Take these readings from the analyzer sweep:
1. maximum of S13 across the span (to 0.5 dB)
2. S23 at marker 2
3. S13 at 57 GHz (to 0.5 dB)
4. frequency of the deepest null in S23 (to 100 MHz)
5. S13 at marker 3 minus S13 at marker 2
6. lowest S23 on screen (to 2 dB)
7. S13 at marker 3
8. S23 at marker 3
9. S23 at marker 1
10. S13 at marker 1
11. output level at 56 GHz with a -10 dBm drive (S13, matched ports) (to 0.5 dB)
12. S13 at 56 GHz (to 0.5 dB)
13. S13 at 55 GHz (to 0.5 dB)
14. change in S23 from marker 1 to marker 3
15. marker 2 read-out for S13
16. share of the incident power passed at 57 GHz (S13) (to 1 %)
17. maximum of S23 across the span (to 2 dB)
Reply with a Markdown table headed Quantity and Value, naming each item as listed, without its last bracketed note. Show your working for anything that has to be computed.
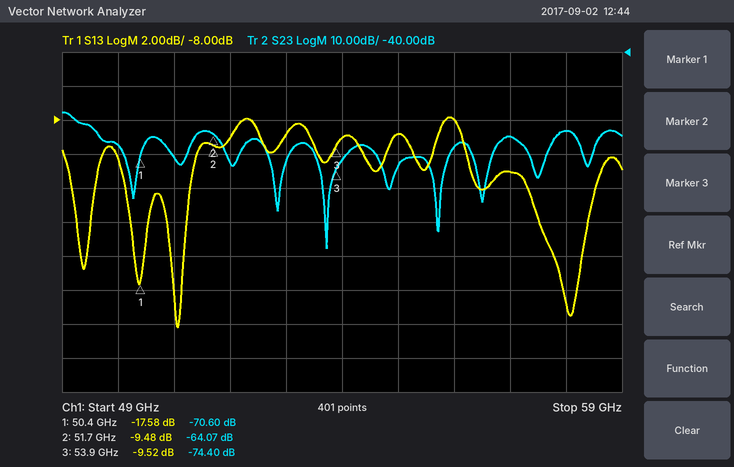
| Quantity | Value |
|---|---|
| maximum of S13 across the span | -8.0 dB |
| S23 at marker 2 | -64.07 dB |
| S13 at 57 GHz | -11.0 dB |
| frequency of the deepest null in S23 | 53.7 GHz |
| S13 at marker 3 minus S13 at marker 2 | -9.52 − (-9.48) = -0.04 dB |
| lowest S23 on screen | -98 dB |
| S13 at marker 3 | -9.52 dB |
| S23 at marker 3 | -74.40 dB |
| S23 at marker 1 | -70.60 dB |
| S13 at marker 1 | -17.58 dB |
| output level at 56 GHz with a -10 dBm drive (S13, matched ports) | -10 dBm + (-8.0 dB) = -18.0 dBm |
| S13 at 56 GHz | -8.0 dB |
| S13 at 55 GHz | -9.0 dB |
| change in S23 from marker 1 to marker 3 | -74.4 − (-70.6) = -3.80 dB |
| marker 2 read-out for S13 | -9.48 dB |
| share of the incident power passed at 57 GHz (S13) | 10^(-11/10) ≈ 8 % |
| maximum of S23 across the span | -58 dB |
